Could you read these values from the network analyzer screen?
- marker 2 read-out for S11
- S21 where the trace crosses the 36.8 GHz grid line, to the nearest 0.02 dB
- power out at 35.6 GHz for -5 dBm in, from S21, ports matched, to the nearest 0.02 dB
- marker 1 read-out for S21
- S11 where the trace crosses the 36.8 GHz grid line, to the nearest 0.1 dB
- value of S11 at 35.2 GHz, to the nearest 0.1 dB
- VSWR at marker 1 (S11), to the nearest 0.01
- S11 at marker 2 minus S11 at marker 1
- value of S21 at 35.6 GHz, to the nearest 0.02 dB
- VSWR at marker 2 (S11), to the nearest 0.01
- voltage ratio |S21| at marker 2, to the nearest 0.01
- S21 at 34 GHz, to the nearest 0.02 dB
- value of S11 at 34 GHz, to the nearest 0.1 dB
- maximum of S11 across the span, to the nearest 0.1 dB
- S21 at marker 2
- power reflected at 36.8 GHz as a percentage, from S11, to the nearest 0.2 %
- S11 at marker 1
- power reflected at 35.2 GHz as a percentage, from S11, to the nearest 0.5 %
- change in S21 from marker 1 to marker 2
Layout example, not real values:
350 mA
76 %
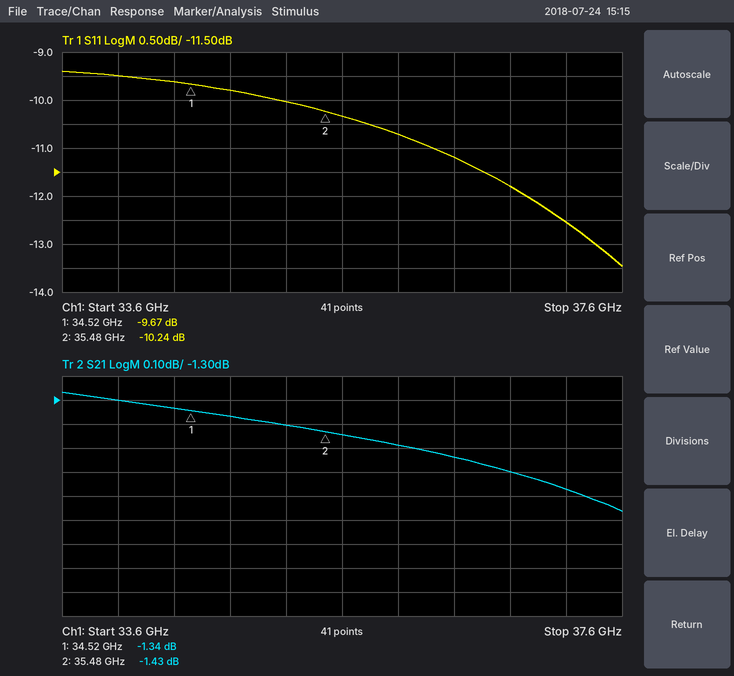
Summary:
-10.24 dB
-1.60 dB
-6.44 dBm
-1.34 dB
-11.8 dB
-10.0 dB
1.98
-0.57 dB
-1.44 dB
1.89
0.85
-1.30 dB
-9.5 dB
-9.4 dB
-1.43 dB
6.6 %
-9.67 dB
10.0 %
-0.09 dB
